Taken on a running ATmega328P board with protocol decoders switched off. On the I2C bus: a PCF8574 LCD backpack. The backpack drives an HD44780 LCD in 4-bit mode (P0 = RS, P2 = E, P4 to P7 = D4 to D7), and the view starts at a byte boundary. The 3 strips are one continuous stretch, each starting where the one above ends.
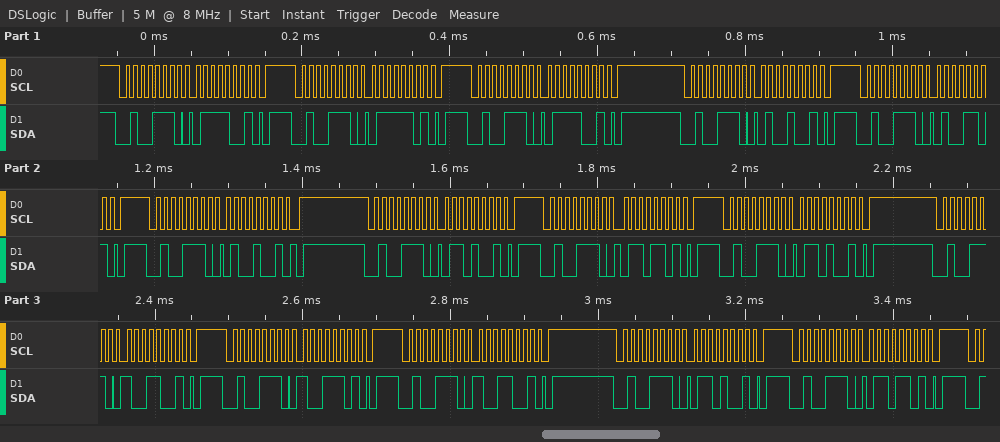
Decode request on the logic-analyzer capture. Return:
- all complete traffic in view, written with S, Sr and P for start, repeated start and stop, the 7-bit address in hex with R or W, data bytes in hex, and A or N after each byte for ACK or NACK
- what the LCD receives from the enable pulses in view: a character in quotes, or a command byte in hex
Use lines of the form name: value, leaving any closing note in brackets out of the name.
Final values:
all complete traffic in view, written with S, Sr and P for start, repeated start and stop, the 7-bit address in hex with R or W, data bytes in hex, and A or N after each byte for ACK or NACK: S 27W A 79 A P S 27W A 7D A P S 27W A 79 A P S 27W A 49 A P S 27W A 4D A P S 27W A 49 A P S 27W A 69 A P S 27W A 6D A P S 27W A 69 A P S 27W A 99 A P S 27W A 9D A P S 27W A 99 A P S 27W A 69 A P S 27W A 6D A P
what the LCD receives from the enable pulses in view: a character in quotes, or a command byte in hex: 't' 'i'
